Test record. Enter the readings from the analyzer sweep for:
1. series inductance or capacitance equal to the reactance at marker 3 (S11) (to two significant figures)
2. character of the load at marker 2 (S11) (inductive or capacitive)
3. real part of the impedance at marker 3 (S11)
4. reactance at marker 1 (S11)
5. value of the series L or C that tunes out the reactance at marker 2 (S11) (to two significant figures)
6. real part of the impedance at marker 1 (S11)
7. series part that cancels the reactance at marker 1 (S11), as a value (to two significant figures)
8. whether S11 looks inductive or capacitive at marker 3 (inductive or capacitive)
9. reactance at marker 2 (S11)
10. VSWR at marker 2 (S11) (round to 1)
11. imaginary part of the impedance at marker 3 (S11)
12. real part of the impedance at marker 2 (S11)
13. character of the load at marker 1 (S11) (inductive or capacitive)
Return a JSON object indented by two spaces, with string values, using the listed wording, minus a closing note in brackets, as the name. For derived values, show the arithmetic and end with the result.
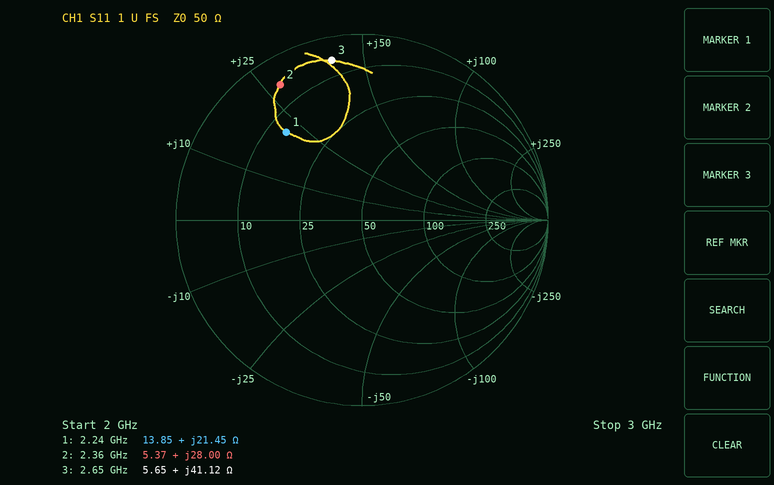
{
  "series inductance or capacitance equal to the reactance at marker 3 (S11)": "L = 41.12 Ω/(2π × 2.65 GHz) ≈ 2.5 nH",
  "character of the load at marker 2 (S11)": "inductive",
  "real part of the impedance at marker 3": "5.65 Ω",
  "reactance at marker 1": "+21.45 Ω",
  "value of the series L or C that tunes out the reactance at marker 2 (S11)": "C = 1/(2π × 2.36 GHz × 28 Ω) ≈ 2.4 pF",
  "real part of the impedance at marker 1": "13.85 Ω",
  "series part that cancels the reactance at marker 1 (S11), as a value": "C = 1/(2π × 2.24 GHz × 21.45 Ω) ≈ 3.3 pF",
  "whether S11 looks inductive or capacitive at marker 3": "inductive",
  "reactance at marker 2": "+28.00 Ω",
  "VSWR at marker 2 (S11)": "12",
  "imaginary part of the impedance at marker 3": "+41.12 Ω",
  "real part of the impedance at marker 2": "5.37 Ω",
  "character of the load at marker 1 (S11)": "inductive"
}
